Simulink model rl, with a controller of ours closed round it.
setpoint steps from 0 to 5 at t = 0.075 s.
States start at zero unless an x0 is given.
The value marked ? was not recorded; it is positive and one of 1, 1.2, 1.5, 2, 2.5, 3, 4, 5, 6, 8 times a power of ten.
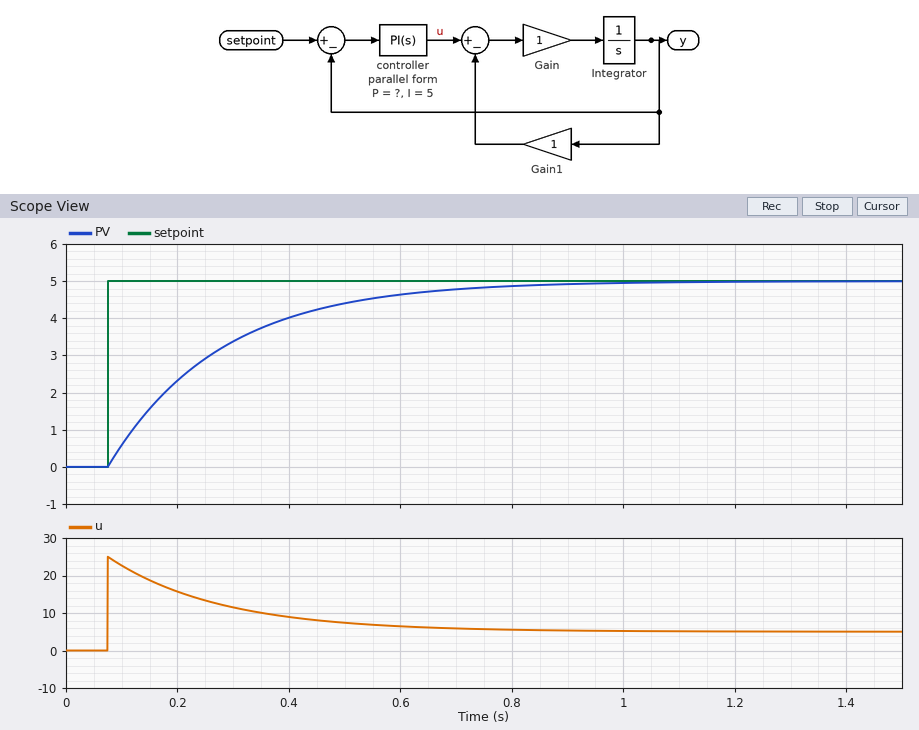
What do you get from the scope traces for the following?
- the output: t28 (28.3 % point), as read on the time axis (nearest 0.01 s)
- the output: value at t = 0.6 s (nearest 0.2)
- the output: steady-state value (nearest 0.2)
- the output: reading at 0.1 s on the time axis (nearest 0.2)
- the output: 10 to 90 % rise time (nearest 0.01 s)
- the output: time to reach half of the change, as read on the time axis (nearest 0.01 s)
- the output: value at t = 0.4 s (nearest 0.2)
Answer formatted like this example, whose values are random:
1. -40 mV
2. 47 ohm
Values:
1. 0.14 s
2. 4.6
3. 5.0
4. 0.6
5. 0.44 s
6. 0.21 s
7. 4.0
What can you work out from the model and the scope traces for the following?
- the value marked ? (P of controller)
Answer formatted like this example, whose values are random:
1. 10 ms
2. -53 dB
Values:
1. 5
